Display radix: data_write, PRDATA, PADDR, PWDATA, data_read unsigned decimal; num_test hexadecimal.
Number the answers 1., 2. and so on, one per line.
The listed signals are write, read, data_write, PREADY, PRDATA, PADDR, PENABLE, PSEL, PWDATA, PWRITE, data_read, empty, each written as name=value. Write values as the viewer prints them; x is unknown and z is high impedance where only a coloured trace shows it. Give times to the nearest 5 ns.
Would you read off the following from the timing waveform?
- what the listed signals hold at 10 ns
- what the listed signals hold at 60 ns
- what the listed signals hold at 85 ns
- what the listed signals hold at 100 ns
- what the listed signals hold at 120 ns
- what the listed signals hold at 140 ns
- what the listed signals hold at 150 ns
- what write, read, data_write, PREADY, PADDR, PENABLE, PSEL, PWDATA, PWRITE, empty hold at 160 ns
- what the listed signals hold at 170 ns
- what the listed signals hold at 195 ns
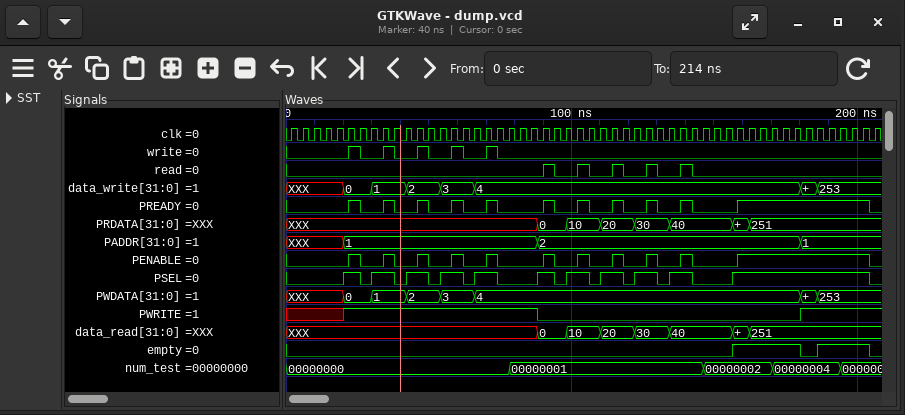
1. write=0, read=0, data_write=XXX, PREADY=0, PRDATA=XXX, PADDR=XXX, PENABLE=0, PSEL=0, PWDATA=XXX, PWRITE=x, data_read=XXX, empty=0
2. write=1, read=0, data_write=3, PREADY=1, PRDATA=XXX, PADDR=1, PENABLE=1, PSEL=1, PWDATA=3, PWRITE=1, data_read=XXX, empty=0
3. write=0, read=0, data_write=4, PREADY=0, PRDATA=XXX, PADDR=1, PENABLE=0, PSEL=0, PWDATA=4, PWRITE=1, data_read=XXX, empty=0
4. write=0, read=0, data_write=4, PREADY=0, PRDATA=10, PADDR=2, PENABLE=0, PSEL=1, PWDATA=4, PWRITE=0, data_read=10, empty=0
5. write=0, read=0, data_write=4, PREADY=0, PRDATA=20, PADDR=2, PENABLE=0, PSEL=0, PWDATA=4, PWRITE=0, data_read=20, empty=0
6. write=0, read=1, data_write=4, PREADY=1, PRDATA=40, PADDR=2, PENABLE=1, PSEL=1, PWDATA=4, PWRITE=0, data_read=40, empty=0
7. write=0, read=0, data_write=4, PREADY=0, PRDATA=40, PADDR=2, PENABLE=0, PSEL=0, PWDATA=4, PWRITE=0, data_read=40, empty=0
8. write=0, read=0, data_write=4, PREADY=1, PADDR=2, PENABLE=1, PSEL=1, PWDATA=4, PWRITE=0, empty=1
9. write=0, read=0, data_write=4, PREADY=1, PRDATA=251, PADDR=2, PENABLE=1, PSEL=1, PWDATA=4, PWRITE=0, data_read=251, empty=1
10. write=0, read=0, data_write=253, PREADY=1, PRDATA=251, PADDR=1, PENABLE=1, PSEL=1, PWDATA=253, PWRITE=1, data_read=251, empty=1
